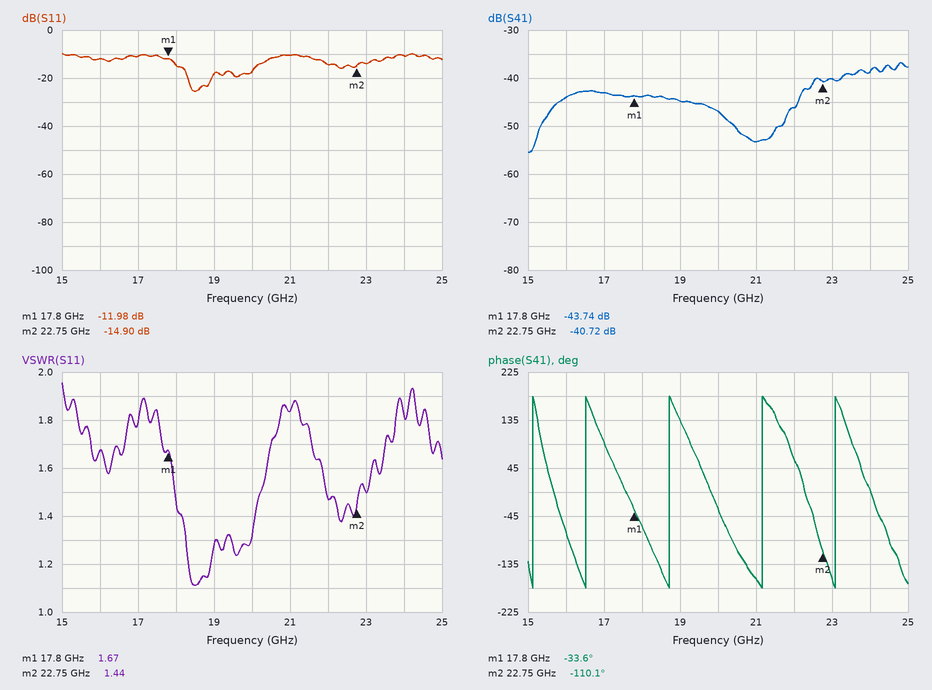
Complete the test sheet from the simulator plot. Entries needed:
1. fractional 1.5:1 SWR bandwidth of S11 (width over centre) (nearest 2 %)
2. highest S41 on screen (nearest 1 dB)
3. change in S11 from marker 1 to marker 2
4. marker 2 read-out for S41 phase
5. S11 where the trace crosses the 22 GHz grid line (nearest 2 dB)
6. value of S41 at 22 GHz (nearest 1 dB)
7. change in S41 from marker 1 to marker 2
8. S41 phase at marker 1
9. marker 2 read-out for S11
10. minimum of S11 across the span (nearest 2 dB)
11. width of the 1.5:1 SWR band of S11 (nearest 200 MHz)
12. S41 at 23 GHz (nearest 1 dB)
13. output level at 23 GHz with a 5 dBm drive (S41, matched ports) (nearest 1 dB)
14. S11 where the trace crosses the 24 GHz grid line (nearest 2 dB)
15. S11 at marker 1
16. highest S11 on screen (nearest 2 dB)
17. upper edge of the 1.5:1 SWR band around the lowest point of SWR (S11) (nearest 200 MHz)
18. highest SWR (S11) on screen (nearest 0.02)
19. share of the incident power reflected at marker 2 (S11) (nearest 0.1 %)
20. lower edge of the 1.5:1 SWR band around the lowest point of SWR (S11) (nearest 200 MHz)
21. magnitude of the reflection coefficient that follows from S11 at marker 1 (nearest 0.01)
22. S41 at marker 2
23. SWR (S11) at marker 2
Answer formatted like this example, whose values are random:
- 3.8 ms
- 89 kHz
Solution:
- 12 %
- -37 dB
- -2.92 dB
- -110.1°
- -14 dB
- -46 dB
- 3.02 dB
- -33.6°
- -14.90 dB
- -26 dB
- 2.2 GHz
- -40 dB
- -35 dBm
- -10 dB
- -11.98 dB
- -10 dB
- 20.2 GHz
- 1.96
- 3.2 %
- 18.0 GHz
- 0.25
- -40.72 dB
- 1.44
